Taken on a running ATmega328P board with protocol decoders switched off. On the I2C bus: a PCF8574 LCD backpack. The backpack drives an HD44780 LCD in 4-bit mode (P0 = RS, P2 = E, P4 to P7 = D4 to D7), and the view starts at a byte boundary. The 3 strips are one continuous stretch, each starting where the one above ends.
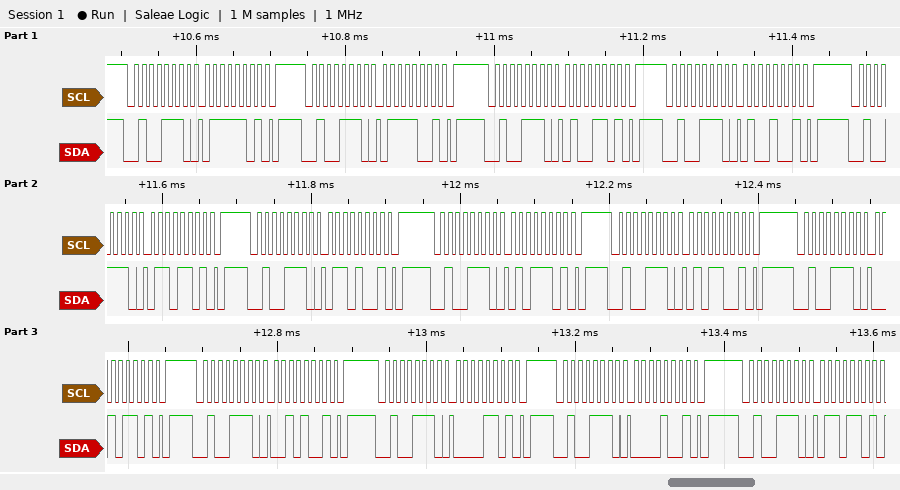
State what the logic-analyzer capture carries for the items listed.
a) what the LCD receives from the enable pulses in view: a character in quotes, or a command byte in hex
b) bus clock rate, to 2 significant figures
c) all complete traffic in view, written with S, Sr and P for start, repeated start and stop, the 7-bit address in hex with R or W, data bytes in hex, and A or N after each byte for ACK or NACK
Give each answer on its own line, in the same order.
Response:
't' 'e' ' '
100 kHz
S 27W A 7D A P S 27W A 79 A P S 27W A 4D A P S 27W A 49 A P S 27W A 6D A P S 27W A 69 A P S 27W A 5D A P S 27W A 59 A P S 27W A 2D A P S 27W A 29 A P S 27W A 0D A P S 27W A 09 A P S 27W A 6D A
